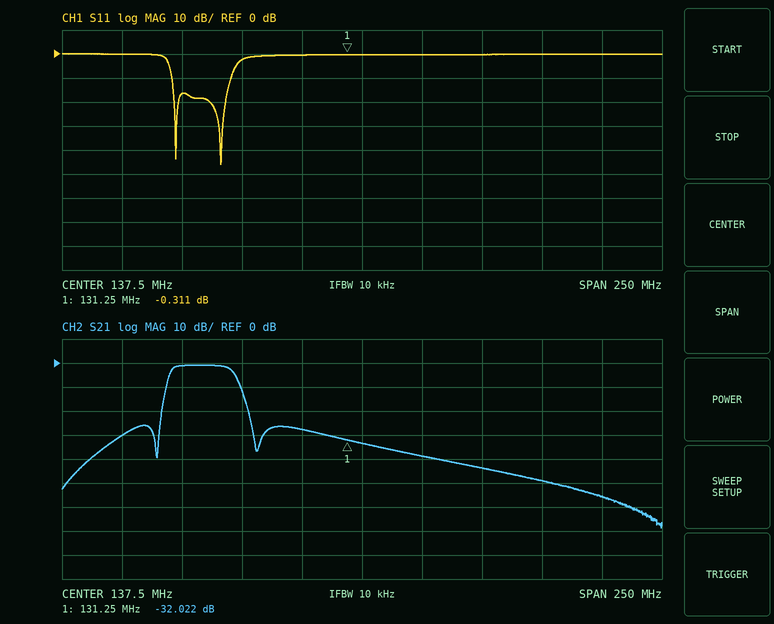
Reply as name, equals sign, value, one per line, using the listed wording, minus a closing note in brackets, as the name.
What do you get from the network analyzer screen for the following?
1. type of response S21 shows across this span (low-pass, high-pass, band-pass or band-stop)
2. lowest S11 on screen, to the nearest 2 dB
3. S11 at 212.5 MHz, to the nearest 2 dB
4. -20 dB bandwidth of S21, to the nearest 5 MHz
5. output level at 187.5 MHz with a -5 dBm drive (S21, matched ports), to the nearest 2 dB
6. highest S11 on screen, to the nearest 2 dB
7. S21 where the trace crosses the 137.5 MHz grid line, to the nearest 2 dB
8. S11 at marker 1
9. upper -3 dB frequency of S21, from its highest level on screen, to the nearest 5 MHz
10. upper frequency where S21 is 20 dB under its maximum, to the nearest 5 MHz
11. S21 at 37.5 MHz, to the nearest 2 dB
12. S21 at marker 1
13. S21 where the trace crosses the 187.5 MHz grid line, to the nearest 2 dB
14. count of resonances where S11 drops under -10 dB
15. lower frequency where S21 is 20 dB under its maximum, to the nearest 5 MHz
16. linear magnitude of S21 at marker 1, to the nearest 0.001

type of response S21 shows across this span = band-pass
lowest S11 on screen, to the nearest 2 dB = -46 dB
S11 at 212.5 MHz, to the nearest 2 dB = 0 dB
-20 dB bandwidth of S21, to the nearest 5 MHz = 35 MHz
output level at 187.5 MHz with a -5 dBm drive (S21, matched ports), to the nearest 2 dB = -48 dBm
highest S11 on screen, to the nearest 2 dB = 0 dB
S21 where the trace crosses the 137.5 MHz grid line, to the nearest 2 dB = -34 dB
S11 at marker 1 = -0.311 dB
upper -3 dB frequency of S21, from its highest level on screen, to the nearest 5 MHz = 85 MHz
upper frequency where S21 is 20 dB under its maximum, to the nearest 5 MHz = 90 MHz
S21 at 37.5 MHz, to the nearest 2 dB = -30 dB
S21 at marker 1 = -32.022 dB
S21 where the trace crosses the 187.5 MHz grid line, to the nearest 2 dB = -44 dB
count of resonances where S11 drops under -10 dB = 2
lower frequency where S21 is 20 dB under its maximum, to the nearest 5 MHz = 55 MHz
linear magnitude of S21 at marker 1, to the nearest 0.001 = 0.025
